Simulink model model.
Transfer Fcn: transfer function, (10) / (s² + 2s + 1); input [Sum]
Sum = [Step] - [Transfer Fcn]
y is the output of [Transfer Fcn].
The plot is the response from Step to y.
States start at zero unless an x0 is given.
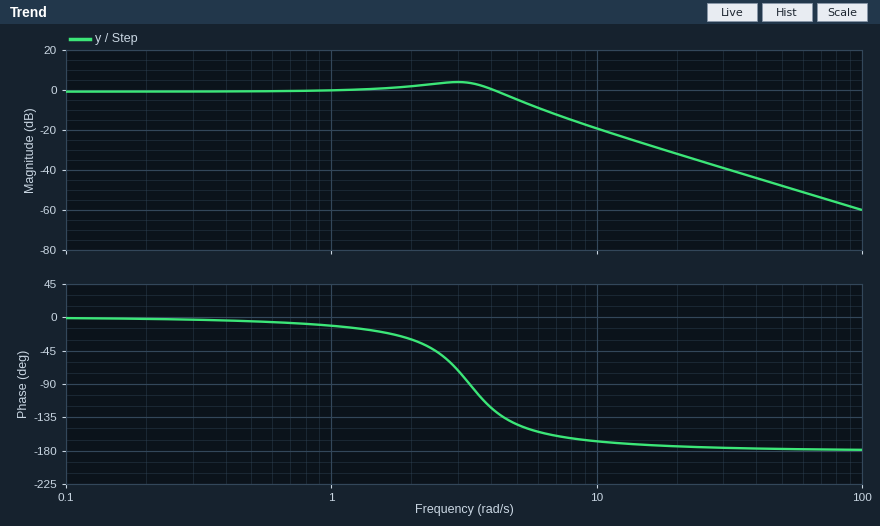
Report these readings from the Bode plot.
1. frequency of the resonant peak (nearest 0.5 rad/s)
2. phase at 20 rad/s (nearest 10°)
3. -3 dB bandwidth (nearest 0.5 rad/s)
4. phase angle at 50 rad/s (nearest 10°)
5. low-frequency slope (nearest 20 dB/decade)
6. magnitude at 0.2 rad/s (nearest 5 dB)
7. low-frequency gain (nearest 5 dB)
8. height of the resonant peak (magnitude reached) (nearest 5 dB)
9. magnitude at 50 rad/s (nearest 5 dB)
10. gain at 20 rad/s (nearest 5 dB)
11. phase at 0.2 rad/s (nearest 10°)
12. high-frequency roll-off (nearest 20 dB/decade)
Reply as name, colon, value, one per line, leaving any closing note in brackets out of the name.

frequency of the resonant peak: 3.0 rad/s
phase at 20 rad/s: -170°
-3 dB bandwidth: 5.0 rad/s
phase angle at 50 rad/s: -180°
low-frequency slope: 0 dB/decade
magnitude at 0.2 rad/s: 0 dB
low-frequency gain: 0 dB
height of the resonant peak (magnitude reached): 5 dB
magnitude at 50 rad/s: -50 dB
gain at 20 rad/s: -30 dB
phase at 0.2 rad/s: 0°
high-frequency roll-off: -40 dB/decade
